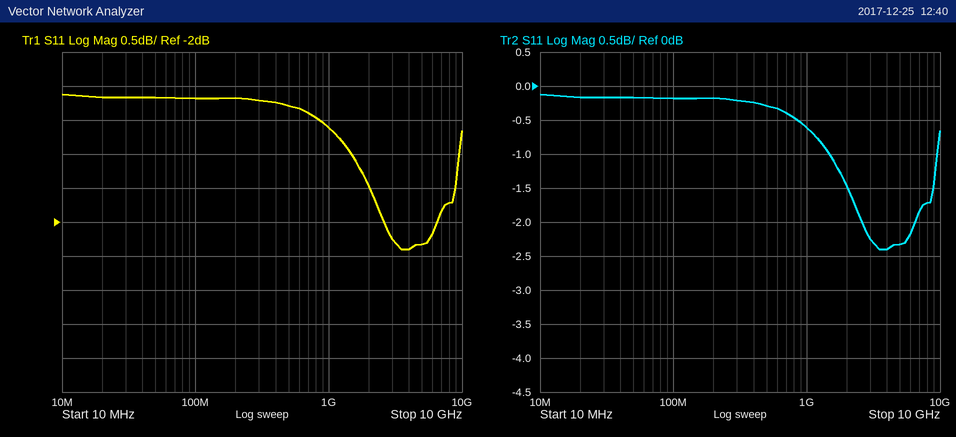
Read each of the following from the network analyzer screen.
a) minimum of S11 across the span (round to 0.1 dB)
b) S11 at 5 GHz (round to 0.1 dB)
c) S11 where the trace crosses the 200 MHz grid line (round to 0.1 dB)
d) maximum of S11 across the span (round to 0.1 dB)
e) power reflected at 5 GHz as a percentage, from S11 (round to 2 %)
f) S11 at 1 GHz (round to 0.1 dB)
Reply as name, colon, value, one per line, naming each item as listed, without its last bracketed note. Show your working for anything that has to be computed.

minimum of S11 across the span: -2.4 dB
S11 at 5 GHz: -2.3 dB
S11 where the trace crosses the 200 MHz grid line: -0.2 dB
maximum of S11 across the span: -0.1 dB
power reflected at 5 GHz as a percentage, from S11: 10^(-2.3/10) ≈ 58.9 %, so 58 % to the nearest 2 %
S11 at 1 GHz: -0.6 dB
